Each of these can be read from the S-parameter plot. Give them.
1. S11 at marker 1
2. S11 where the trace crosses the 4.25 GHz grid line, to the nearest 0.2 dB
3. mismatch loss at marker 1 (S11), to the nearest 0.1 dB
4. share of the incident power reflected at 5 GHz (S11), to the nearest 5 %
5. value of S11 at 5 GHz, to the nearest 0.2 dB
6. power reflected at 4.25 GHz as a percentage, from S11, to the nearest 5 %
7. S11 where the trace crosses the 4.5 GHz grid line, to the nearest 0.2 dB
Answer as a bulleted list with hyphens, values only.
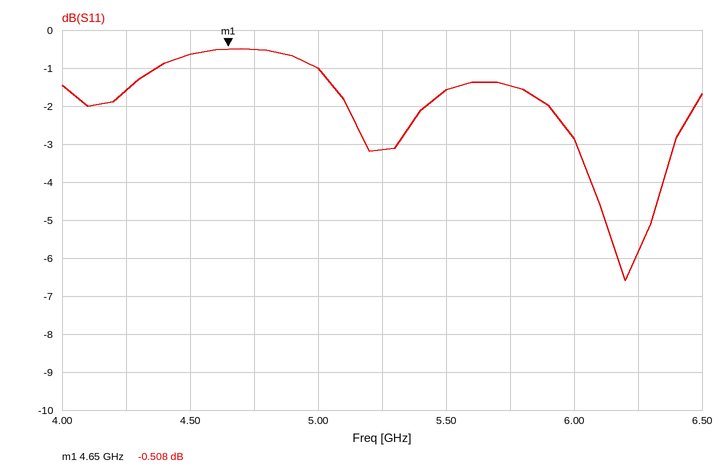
- -0.508 dB
- -1.6 dB
- 9.6 dB
- 80 %
- -1.0 dB
- 70 %
- -0.6 dB
